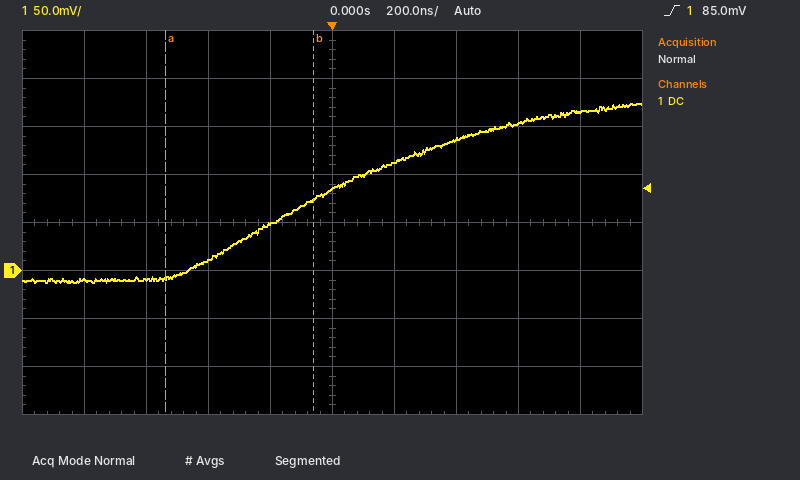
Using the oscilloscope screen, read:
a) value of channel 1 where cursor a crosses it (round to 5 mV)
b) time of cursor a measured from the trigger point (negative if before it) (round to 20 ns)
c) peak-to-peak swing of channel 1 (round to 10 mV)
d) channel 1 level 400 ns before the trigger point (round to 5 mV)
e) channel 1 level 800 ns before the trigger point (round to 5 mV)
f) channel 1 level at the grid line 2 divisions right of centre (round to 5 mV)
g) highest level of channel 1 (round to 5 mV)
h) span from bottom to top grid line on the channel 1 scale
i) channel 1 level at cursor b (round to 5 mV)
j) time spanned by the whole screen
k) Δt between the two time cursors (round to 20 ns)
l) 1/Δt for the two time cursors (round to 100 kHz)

-10 mV
-540 ns
190 mV
10 mV
-10 mV
135 mV
175 mV
400 mV
75 mV
2 µs
480 ns
2.1 MHz
